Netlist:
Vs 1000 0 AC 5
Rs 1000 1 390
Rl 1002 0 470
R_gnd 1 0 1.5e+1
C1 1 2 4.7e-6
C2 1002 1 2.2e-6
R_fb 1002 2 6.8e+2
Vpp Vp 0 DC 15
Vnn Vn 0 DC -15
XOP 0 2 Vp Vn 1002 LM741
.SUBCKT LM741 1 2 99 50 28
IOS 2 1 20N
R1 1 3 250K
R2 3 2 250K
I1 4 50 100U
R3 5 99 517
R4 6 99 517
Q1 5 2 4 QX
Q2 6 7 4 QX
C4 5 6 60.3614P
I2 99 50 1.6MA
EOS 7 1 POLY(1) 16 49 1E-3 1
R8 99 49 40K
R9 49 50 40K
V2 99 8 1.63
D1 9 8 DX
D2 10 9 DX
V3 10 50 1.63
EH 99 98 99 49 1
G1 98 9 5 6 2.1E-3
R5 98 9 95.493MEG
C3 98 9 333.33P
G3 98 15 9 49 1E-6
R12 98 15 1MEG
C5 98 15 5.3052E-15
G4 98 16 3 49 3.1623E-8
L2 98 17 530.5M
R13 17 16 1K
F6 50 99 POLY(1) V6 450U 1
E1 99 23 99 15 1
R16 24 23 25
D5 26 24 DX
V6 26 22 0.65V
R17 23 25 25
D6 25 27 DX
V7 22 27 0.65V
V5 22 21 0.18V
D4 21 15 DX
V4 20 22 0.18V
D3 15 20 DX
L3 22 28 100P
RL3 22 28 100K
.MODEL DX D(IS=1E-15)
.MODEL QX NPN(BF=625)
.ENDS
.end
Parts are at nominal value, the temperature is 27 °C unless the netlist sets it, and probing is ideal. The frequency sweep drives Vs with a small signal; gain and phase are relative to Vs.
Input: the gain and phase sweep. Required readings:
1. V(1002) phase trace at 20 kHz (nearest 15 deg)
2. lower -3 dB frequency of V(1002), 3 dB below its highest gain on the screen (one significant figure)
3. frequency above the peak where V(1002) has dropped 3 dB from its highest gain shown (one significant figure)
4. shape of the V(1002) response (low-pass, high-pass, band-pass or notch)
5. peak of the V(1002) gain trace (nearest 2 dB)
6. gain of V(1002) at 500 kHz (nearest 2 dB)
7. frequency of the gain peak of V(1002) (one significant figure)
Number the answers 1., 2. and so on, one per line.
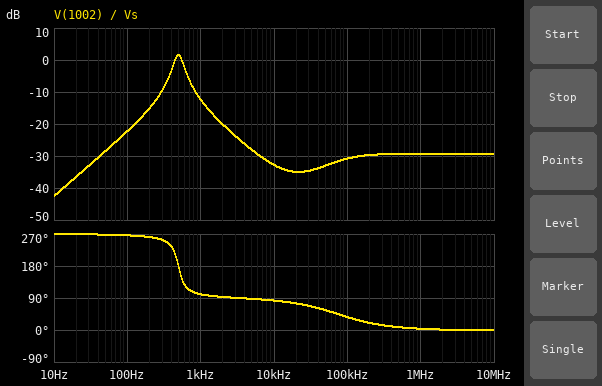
1. 75 deg
2. 400 Hz
3. 600 Hz
4. band-pass
5. 2 dB
6. -30 dB
7. 500 Hz
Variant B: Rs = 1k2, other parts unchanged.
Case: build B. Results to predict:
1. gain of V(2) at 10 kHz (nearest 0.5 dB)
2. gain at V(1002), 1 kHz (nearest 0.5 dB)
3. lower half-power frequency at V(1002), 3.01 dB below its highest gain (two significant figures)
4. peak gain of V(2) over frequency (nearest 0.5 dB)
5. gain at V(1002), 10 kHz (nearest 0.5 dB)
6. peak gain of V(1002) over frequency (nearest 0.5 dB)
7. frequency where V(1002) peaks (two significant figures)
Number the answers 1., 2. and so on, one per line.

1. -56.5 dB
2. -22.0 dB
3. 420 Hz
4. -39.0 dB
5. -42.5 dB
6. -8.0 dB
7. 490 Hz
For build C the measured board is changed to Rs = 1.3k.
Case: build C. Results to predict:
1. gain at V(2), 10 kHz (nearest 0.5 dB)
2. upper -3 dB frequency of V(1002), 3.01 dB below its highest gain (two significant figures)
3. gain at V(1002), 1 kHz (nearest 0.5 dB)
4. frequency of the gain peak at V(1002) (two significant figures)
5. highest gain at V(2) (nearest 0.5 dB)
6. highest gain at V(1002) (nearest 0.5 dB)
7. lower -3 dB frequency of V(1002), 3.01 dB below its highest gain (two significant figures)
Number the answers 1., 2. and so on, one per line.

1. -57.0 dB
2. 570 Hz
3. -23.0 dB
4. 490 Hz
5. -39.5 dB
6. -9.0 dB
7. 420 Hz
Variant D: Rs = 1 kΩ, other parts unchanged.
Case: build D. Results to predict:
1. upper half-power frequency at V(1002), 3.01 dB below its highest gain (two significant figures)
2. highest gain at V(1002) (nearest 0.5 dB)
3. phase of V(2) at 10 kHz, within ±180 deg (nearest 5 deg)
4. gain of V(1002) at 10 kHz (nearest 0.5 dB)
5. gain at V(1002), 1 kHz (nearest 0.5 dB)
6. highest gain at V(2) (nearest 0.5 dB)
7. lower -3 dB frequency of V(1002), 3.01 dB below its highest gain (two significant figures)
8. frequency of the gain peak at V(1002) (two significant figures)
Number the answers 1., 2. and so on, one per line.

1. 570 Hz
2. -6.5 dB
3. 80 deg
4. -41.0 dB
5. -20.5 dB
6. -37.5 dB
7. 420 Hz
8. 490 Hz
